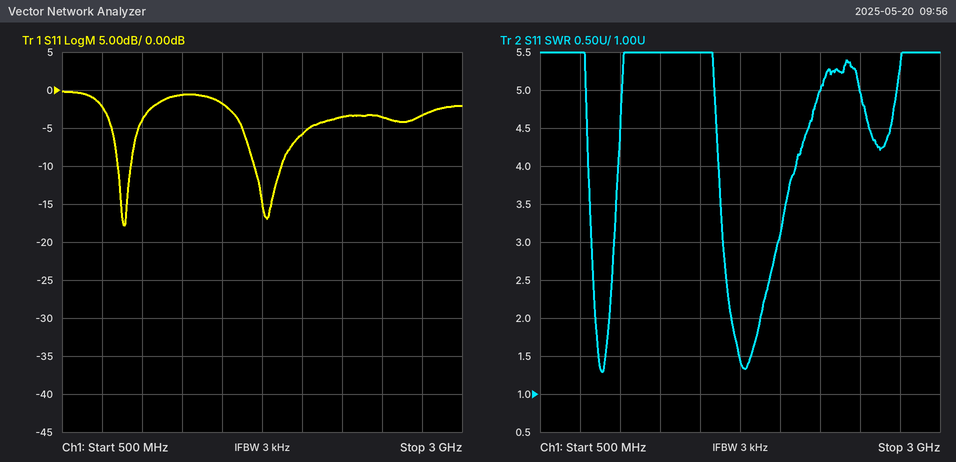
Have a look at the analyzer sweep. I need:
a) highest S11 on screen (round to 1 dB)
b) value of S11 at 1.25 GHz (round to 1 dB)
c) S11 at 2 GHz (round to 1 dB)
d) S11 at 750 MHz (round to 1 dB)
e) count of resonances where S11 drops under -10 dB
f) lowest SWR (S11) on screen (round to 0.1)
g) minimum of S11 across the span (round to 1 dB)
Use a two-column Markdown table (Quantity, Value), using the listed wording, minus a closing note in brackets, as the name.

| Quantity | Value |
|---|---|
| highest S11 on screen | 0 dB |
| value of S11 at 1.25 GHz | -1 dB |
| S11 at 2 GHz | -6 dB |
| S11 at 750 MHz | -2 dB |
| count of resonances where S11 drops under -10 dB | 2 |
| lowest SWR (S11) on screen | 1.3 |
| minimum of S11 across the span | -18 dB |
